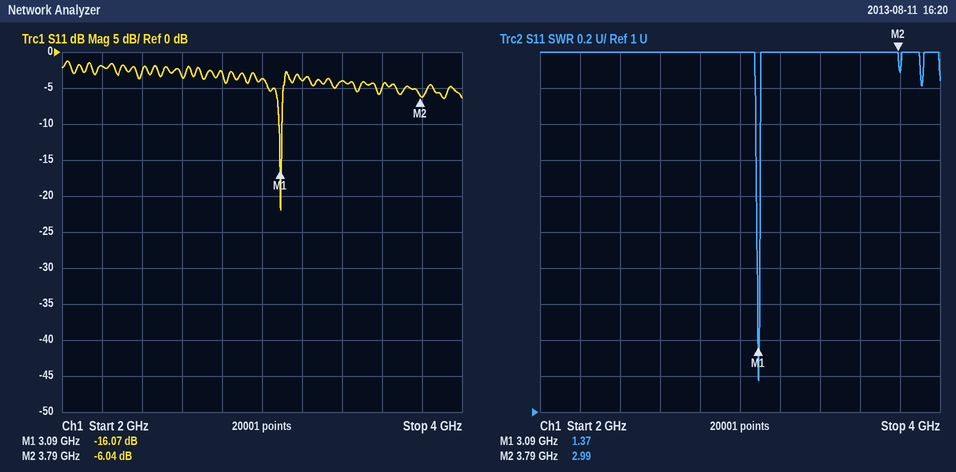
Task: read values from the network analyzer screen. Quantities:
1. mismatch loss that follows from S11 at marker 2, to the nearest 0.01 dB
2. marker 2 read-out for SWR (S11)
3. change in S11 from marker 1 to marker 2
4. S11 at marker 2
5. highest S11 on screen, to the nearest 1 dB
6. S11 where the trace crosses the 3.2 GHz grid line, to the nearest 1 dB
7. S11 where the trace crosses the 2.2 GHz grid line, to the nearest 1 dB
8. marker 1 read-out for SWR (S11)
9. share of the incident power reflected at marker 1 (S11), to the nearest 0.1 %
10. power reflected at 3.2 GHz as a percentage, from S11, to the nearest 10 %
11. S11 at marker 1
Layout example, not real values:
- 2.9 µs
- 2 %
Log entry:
- 1.24 dB
- 2.99
- 10.03 dB
- -6.04 dB
- -1 dB
- -4 dB
- -2 dB
- 1.37
- 2.5 %
- 40 %
- -16.07 dB
